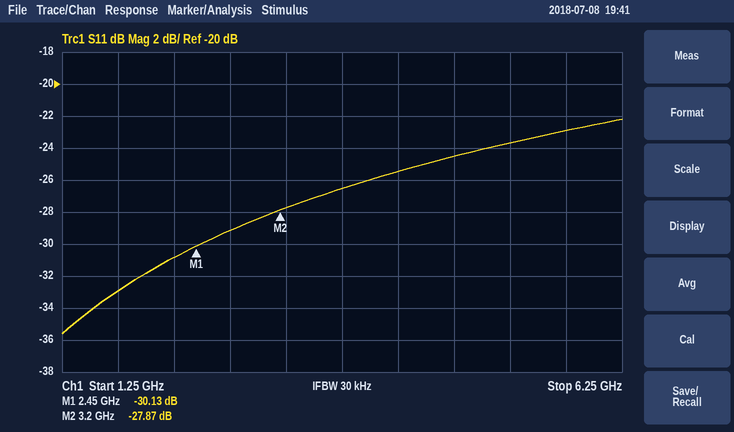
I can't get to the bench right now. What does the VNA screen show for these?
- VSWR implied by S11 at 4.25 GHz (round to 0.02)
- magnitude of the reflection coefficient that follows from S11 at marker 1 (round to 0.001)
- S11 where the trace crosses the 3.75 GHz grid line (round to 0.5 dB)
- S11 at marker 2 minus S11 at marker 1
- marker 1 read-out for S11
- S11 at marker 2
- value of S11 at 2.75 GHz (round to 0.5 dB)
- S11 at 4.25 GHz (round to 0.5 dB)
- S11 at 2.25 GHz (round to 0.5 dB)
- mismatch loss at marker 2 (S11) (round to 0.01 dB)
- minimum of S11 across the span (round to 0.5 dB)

1.12
0.031
-26.5 dB
2.26 dB
-30.13 dB
-27.87 dB
-29.0 dB
-25.5 dB
-31.0 dB
0.01 dB
-35.5 dB
